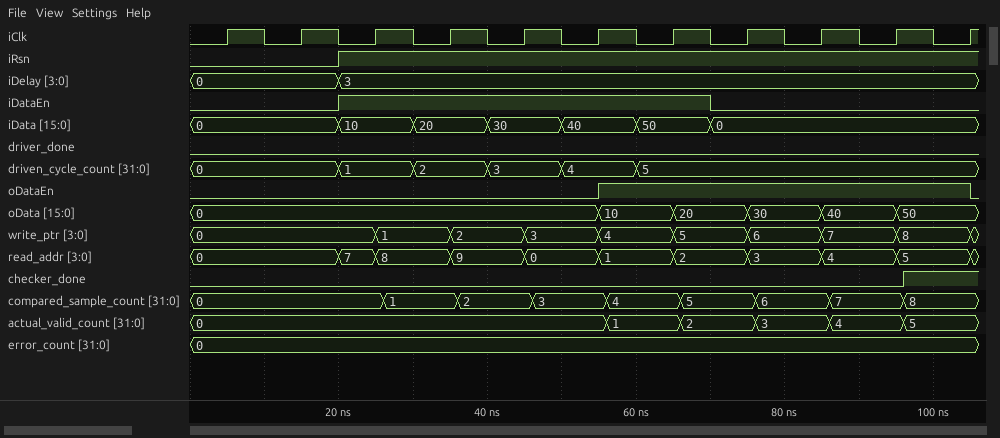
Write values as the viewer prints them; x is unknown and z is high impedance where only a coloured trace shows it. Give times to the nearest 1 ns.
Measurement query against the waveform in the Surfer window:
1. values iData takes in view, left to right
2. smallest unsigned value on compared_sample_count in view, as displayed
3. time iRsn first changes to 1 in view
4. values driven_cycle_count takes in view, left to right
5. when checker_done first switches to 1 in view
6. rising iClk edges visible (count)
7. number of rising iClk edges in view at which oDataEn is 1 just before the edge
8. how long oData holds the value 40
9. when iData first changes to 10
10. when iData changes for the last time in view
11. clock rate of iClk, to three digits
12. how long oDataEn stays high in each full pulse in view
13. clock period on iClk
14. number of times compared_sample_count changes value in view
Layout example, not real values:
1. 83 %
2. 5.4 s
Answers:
1. 0, 10, 20, 30, 40, 50, 0
2. 0
3. 20 ns
4. 0, 1, 2, 3, 4, 5
5. 96 ns
6. 11
7. 5
8. 10 ns
9. 20 ns
10. 70 ns
11. 100 MHz
12. 50 ns
13. 10 ns
14. 8
